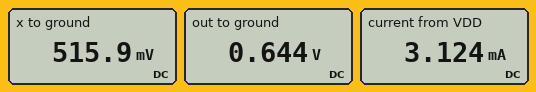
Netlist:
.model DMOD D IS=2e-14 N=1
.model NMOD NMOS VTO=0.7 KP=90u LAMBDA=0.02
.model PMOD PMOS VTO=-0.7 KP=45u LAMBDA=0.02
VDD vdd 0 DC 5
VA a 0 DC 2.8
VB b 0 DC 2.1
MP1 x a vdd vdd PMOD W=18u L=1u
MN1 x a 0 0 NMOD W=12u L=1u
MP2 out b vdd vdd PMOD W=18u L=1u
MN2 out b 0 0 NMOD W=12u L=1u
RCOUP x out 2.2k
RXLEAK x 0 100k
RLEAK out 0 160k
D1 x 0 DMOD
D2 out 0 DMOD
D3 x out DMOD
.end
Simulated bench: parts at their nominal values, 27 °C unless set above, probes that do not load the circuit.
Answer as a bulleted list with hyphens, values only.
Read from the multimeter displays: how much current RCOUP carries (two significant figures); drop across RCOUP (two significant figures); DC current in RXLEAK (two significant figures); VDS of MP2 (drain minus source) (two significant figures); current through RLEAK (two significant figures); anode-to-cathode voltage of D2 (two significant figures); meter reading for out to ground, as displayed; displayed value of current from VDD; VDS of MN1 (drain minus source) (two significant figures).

- 58 µA
- 130 mV
- 5.2 µA
- -4.4 V
- 4.0 µA
- 640 mV
- 0.644 V
- 3.124 mA
- 520 mV
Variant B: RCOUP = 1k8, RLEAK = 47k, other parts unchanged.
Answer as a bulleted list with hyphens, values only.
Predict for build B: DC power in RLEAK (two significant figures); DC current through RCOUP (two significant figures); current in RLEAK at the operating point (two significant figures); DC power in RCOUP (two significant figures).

- 8.8 µW
- 68 µA
- 14 µA
- 8.4 µW
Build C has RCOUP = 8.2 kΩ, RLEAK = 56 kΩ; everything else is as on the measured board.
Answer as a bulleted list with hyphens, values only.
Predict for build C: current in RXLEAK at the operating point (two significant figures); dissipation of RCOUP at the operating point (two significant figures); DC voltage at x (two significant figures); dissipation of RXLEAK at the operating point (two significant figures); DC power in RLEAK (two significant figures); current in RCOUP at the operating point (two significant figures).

- 5.0 µA
- 2.7 µW
- 500 mV
- 2.5 µW
- 7.4 µW
- 18 µA
